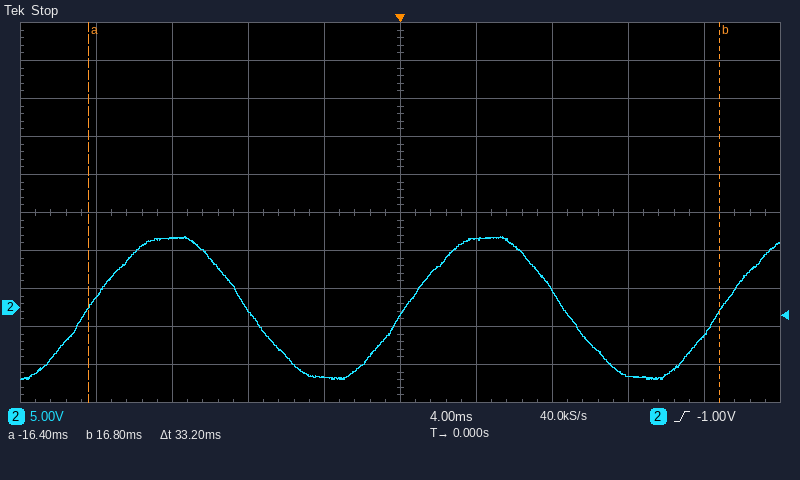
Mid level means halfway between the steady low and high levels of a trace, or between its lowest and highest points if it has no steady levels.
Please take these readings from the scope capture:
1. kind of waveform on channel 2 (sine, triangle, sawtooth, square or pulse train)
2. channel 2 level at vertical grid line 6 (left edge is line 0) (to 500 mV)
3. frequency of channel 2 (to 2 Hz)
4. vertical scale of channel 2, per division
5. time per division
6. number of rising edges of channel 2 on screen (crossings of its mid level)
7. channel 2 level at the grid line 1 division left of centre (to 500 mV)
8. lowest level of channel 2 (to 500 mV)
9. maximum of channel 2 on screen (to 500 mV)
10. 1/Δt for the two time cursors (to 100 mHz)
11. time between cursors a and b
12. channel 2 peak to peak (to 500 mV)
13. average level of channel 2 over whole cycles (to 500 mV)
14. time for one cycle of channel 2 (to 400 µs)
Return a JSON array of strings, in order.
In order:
["sine", "9.0 V", "60 Hz", "5 V", "4 ms", "3", "-9.0 V", "-9.5 V", "9.5 V", "30.1 Hz", "33.2 ms", "19.0 V", "0.0 V", "16.8 ms"]
